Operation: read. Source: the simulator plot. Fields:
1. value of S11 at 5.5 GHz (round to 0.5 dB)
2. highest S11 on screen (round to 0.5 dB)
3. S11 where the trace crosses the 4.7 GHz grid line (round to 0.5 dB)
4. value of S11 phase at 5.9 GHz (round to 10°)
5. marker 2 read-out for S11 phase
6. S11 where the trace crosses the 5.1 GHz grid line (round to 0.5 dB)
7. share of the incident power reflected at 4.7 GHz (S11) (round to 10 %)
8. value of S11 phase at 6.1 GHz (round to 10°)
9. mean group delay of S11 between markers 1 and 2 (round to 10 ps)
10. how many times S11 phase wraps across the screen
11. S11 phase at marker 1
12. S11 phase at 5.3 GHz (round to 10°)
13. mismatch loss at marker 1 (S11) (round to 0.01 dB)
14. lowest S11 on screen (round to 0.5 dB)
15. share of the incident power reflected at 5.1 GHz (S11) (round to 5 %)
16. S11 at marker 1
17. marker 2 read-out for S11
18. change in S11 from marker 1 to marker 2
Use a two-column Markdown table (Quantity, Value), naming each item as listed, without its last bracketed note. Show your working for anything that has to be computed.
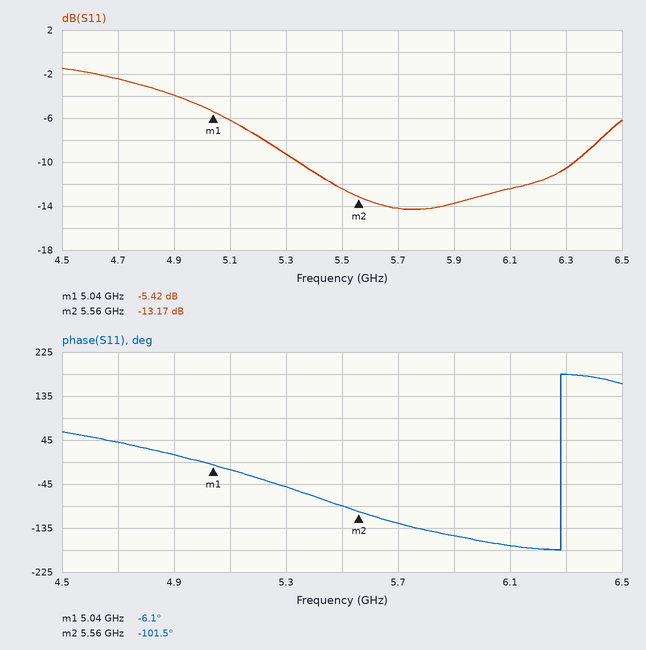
| Quantity | Value |
|---|---|
| value of S11 at 5.5 GHz | -12.5 dB |
| highest S11 on screen | -1.5 dB |
| S11 where the trace crosses the 4.7 GHz grid line | -2.5 dB |
| value of S11 phase at 5.9 GHz | -150° |
| marker 2 read-out for S11 phase | -101.5° |
| S11 where the trace crosses the 5.1 GHz grid line | -6.0 dB |
| share of the incident power reflected at 4.7 GHz (S11) | 10^(-2.5/10) ≈ 56.2 %, so 60 % to the nearest 10 % |
| value of S11 phase at 6.1 GHz | -170° |
| mean group delay of S11 between markers 1 and 2 | −(-101.5° − (-6.1°))/(360° × 520 MHz) ≈ 510 ps |
| how many times S11 phase wraps across the screen | 1 |
| S11 phase at marker 1 | -6.1° |
| S11 phase at 5.3 GHz | -50° |
| mismatch loss at marker 1 (S11) | −10 log10(1 − 10^(-5.42/10)) ≈ 1.47 dB |
| lowest S11 on screen | -14.5 dB |
| share of the incident power reflected at 5.1 GHz (S11) | 10^(-6/10) ≈ 25 % |
| S11 at marker 1 | -5.42 dB |
| marker 2 read-out for S11 | -13.17 dB |
| change in S11 from marker 1 to marker 2 | -13.17 − (-5.42) = -7.75 dB |
